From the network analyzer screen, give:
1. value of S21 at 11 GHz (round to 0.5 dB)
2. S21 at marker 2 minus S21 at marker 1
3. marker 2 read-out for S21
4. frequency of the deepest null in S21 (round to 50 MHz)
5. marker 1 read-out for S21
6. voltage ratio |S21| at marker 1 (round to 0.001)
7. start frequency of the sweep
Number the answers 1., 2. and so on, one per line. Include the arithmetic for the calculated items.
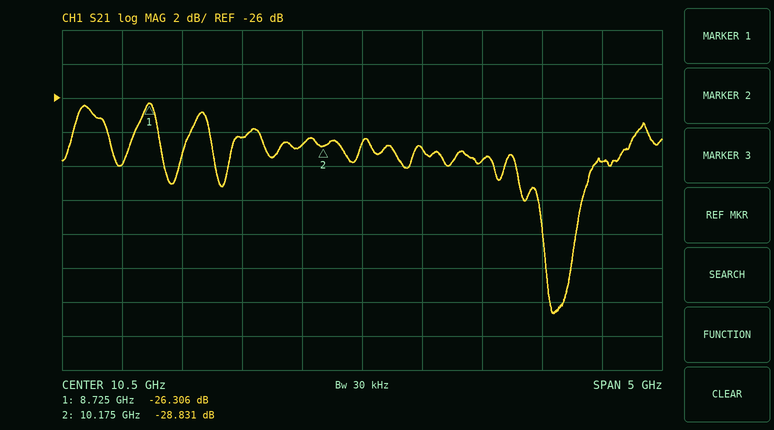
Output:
1. -29.0 dB
2. -28.831 − (-26.306) = -2.525 dB
3. -28.831 dB
4. 12.10 GHz
5. -26.306 dB
6. 10^(-26.306/20) ≈ 0.048
7. 8 GHz
